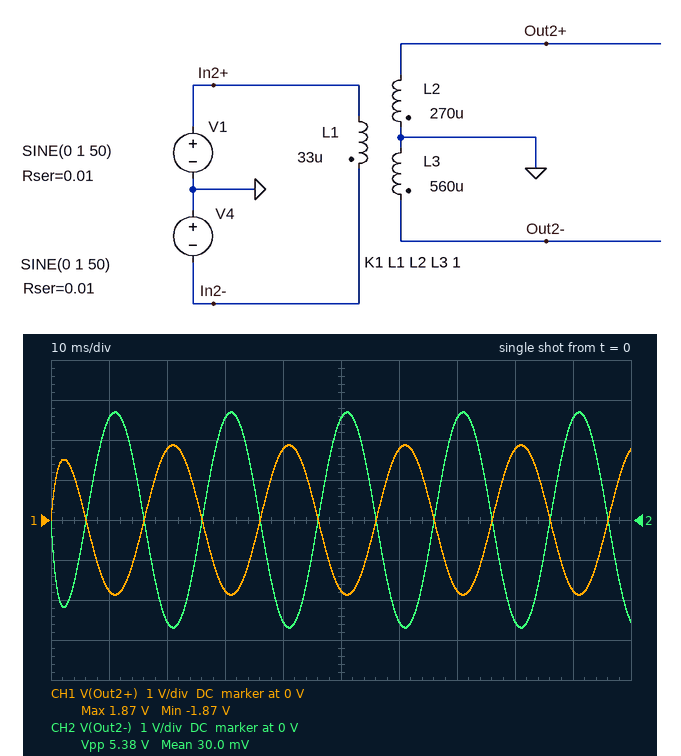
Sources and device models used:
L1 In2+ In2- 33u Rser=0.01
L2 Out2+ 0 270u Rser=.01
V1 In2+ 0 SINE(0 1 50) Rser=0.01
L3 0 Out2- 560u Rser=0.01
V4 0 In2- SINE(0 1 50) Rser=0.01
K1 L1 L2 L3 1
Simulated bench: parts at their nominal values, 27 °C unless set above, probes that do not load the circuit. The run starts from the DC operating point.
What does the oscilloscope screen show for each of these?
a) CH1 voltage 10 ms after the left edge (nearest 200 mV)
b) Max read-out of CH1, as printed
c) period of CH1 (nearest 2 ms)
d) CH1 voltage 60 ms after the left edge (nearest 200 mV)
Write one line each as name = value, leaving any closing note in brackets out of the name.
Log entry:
CH1 voltage 10 ms after the left edge = -1.8 V
Max read-out of CH1, as printed = 1.87 V
period of CH1 = 20 ms
CH1 voltage 60 ms after the left edge = 1.8 V
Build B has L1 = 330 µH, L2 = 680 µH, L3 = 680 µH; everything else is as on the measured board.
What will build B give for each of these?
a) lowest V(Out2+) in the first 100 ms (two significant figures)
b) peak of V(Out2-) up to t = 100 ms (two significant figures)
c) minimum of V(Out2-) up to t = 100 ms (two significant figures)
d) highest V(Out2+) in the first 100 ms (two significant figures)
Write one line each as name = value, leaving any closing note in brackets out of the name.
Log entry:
lowest V(Out2+) in the first 100 ms = -3.0 V
peak of V(Out2-) up to t = 100 ms = 3.0 V
minimum of V(Out2-) up to t = 100 ms = -2.8 V
highest V(Out2+) in the first 100 ms = 2.8 V
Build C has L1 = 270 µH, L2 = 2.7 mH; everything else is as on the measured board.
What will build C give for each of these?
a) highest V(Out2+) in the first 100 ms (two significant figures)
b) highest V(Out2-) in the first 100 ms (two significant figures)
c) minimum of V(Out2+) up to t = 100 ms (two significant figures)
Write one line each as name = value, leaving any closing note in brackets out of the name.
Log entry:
highest V(Out2+) in the first 100 ms = 6.0 V
highest V(Out2-) in the first 100 ms = 2.9 V
minimum of V(Out2+) up to t = 100 ms = -6.4 V
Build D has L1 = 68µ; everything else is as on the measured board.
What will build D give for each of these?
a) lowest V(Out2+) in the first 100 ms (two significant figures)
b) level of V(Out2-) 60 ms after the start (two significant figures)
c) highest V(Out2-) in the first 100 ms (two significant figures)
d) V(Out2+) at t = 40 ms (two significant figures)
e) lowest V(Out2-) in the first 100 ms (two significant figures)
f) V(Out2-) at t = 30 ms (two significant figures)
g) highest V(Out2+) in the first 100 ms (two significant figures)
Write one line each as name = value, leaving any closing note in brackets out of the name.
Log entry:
lowest V(Out2+) in the first 100 ms = -2.3 V
level of V(Out2-) 60 ms after the start = -2.7 V
highest V(Out2-) in the first 100 ms = 3.3 V
V(Out2+) at t = 40 ms = 1.9 V
lowest V(Out2-) in the first 100 ms = -3.3 V
V(Out2-) at t = 30 ms = 2.7 V
highest V(Out2+) in the first 100 ms = 2.3 V
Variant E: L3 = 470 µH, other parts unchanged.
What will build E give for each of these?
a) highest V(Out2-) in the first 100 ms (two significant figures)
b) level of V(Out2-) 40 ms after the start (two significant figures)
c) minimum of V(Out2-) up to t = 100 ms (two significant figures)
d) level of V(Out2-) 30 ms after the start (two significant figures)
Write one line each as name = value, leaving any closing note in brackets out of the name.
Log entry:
highest V(Out2-) in the first 100 ms = 2.5 V
level of V(Out2-) 40 ms after the start = -2.3 V
minimum of V(Out2-) up to t = 100 ms = -2.5 V
level of V(Out2-) 30 ms after the start = 2.3 V
